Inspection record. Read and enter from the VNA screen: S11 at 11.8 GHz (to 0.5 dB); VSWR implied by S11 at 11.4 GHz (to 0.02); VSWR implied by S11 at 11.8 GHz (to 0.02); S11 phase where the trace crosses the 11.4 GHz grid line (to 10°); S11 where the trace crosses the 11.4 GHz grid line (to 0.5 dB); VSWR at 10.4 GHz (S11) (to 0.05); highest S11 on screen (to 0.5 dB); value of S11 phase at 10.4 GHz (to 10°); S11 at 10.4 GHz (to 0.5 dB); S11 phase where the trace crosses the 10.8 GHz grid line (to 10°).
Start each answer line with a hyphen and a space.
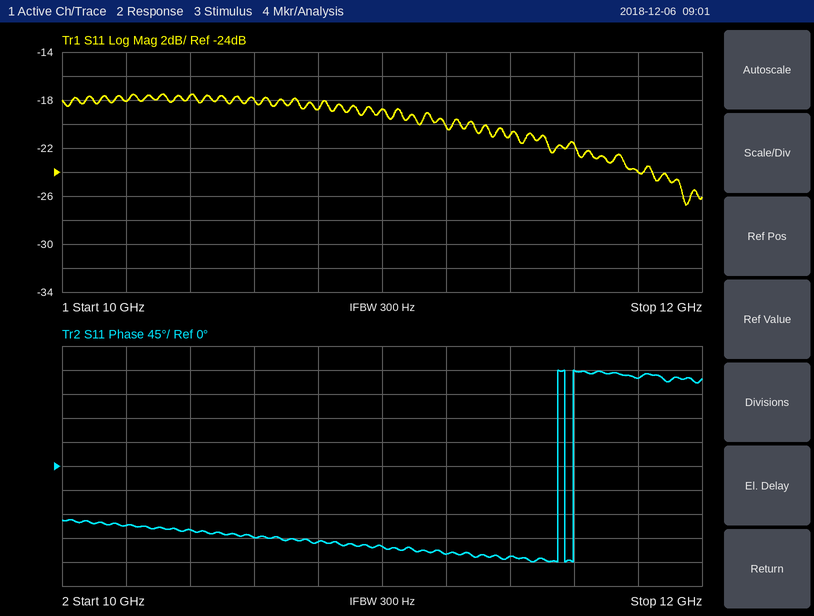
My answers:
- -24.0 dB
- 1.20
- 1.14
- -170°
- -21.0 dB
- 1.30
- -17.5 dB
- -120°
- -17.5 dB
- -140°
